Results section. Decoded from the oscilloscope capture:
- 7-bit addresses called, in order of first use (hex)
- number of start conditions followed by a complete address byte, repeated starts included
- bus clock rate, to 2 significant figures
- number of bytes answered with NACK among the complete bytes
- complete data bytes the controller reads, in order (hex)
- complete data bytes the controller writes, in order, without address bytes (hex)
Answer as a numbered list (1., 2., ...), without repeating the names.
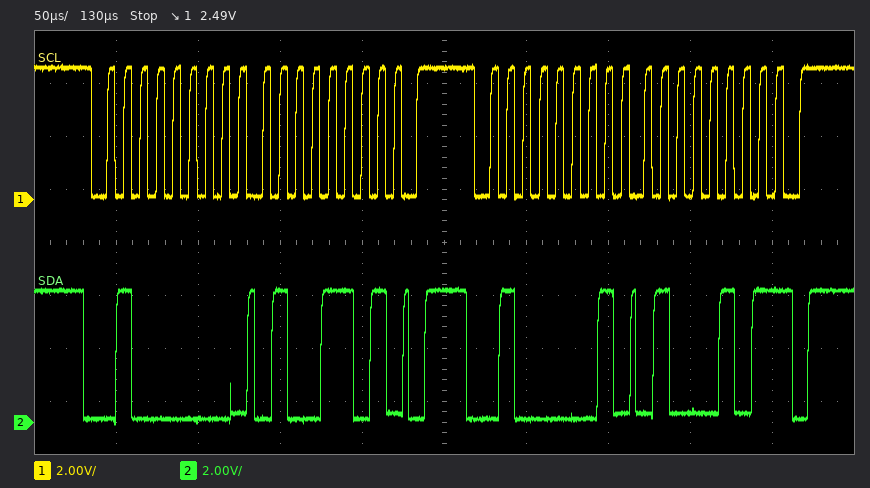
1. 0x20
2. 2
3. 100 kHz
4. 1
5. 45
6. 4D
